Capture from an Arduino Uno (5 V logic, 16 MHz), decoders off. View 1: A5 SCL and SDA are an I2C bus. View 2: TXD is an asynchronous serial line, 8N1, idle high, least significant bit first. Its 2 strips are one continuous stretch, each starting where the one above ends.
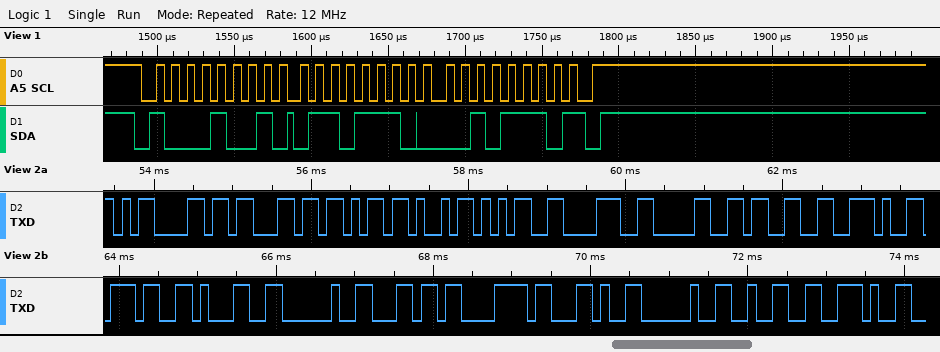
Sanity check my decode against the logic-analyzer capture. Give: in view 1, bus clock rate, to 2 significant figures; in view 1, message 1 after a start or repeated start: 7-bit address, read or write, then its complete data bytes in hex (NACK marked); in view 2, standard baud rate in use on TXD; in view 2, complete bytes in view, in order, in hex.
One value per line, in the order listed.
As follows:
100 kHz
0x44 read: 6E 2E NACK
9600 baud
0D 1B 5B 4B 35 38 30 33 2E 37 31 20 6C 78 2C 20 32 2E
